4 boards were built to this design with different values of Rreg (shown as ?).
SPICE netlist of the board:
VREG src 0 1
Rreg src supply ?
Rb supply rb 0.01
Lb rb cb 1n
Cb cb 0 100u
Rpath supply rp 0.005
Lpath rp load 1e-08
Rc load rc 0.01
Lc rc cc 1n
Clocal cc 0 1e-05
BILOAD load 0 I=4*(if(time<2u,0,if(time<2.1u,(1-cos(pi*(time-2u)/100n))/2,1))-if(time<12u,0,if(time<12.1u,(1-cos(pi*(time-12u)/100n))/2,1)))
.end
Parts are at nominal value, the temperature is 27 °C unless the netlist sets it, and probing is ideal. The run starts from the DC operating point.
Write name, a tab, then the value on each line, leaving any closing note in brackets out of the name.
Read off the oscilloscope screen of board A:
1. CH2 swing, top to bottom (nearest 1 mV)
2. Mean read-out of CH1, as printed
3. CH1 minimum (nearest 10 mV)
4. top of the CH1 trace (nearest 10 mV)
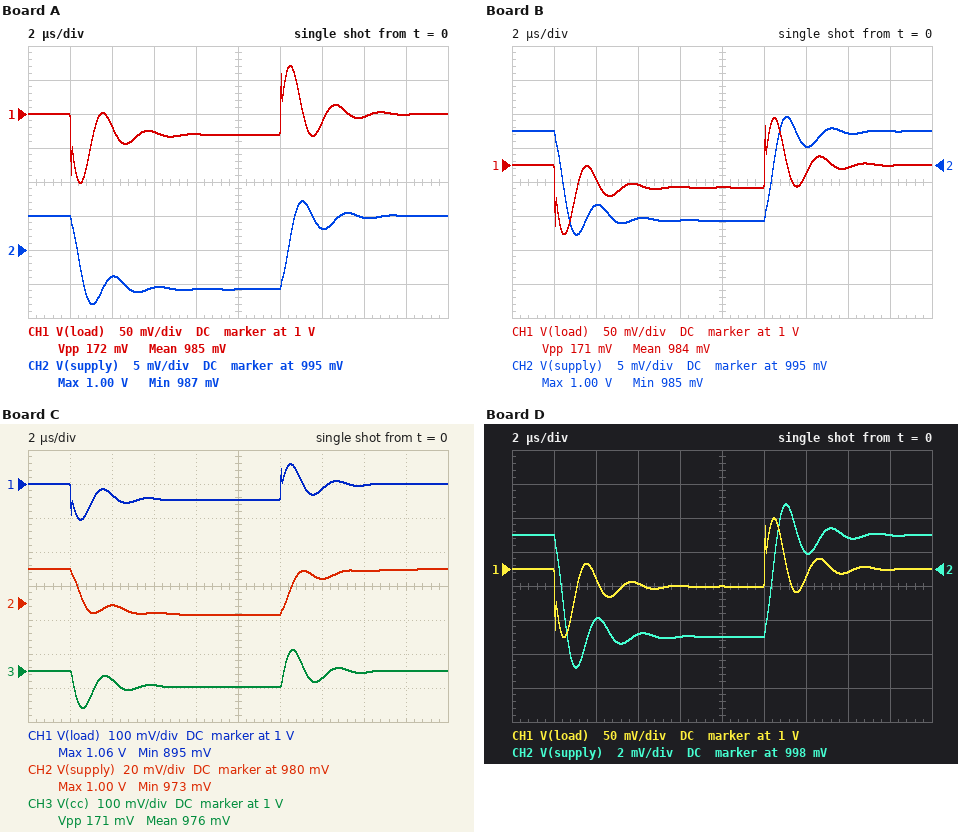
CH2 swing, top to bottom	15 mV
Mean read-out of CH1, as printed	985 mV
CH1 minimum	900 mV
top of the CH1 trace	1.07 V
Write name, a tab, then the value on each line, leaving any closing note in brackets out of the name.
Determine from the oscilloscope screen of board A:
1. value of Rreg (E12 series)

value of Rreg	2.7 mΩ
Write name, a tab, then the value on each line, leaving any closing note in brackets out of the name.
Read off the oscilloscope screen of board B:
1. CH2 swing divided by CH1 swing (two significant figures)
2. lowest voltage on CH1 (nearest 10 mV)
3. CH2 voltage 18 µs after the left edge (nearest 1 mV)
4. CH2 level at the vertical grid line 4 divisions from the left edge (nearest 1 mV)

CH2 swing divided by CH1 swing	0.10
lowest voltage on CH1	900 mV
CH2 voltage 18 µs after the left edge	1.000 V
CH2 level at the vertical grid line 4 divisions from the left edge	987 mV
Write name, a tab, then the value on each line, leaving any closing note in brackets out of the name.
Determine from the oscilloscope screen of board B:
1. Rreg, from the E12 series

Rreg, from the E12 series	3.3 mΩ
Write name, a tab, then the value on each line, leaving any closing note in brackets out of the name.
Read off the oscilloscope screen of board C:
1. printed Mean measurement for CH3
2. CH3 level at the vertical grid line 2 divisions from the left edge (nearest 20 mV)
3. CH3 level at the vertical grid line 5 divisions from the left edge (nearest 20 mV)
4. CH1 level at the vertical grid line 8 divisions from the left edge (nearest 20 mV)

printed Mean measurement for CH3	976 mV
CH3 level at the vertical grid line 2 divisions from the left edge	980 mV
CH3 level at the vertical grid line 5 divisions from the left edge	960 mV
CH1 level at the vertical grid line 8 divisions from the left edge	1.00 V
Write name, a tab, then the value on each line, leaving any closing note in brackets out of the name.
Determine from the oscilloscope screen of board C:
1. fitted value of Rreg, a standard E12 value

fitted value of Rreg, a standard E12 value	6.8 mΩ
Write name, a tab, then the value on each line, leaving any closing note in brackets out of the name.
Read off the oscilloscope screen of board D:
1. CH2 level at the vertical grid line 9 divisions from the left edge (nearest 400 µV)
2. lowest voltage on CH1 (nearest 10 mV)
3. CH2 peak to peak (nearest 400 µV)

CH2 level at the vertical grid line 9 divisions from the left edge	1.0000 V
lowest voltage on CH1	900 mV
CH2 peak to peak	9.6 mV
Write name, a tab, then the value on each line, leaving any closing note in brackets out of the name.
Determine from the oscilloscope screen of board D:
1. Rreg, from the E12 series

Rreg, from the E12 series	1.5 mΩ
